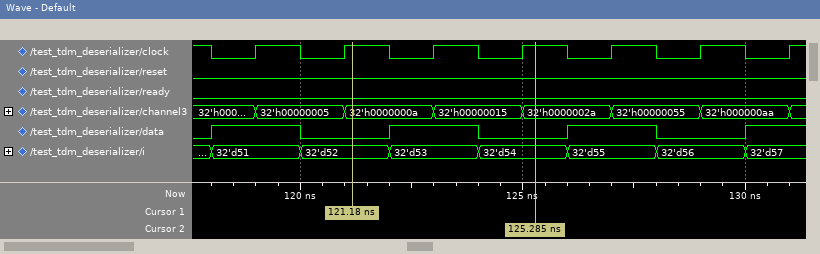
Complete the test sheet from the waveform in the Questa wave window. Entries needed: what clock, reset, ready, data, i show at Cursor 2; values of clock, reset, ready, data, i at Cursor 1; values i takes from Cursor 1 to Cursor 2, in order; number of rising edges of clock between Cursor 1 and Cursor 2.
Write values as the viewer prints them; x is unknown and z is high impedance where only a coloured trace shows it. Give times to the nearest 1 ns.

clock=1, reset=0, ready=0, data=0, i=32'd54
clock=1, reset=0, ready=0, data=0, i=32'd52
32'd52, 32'd53, 32'd54
2
